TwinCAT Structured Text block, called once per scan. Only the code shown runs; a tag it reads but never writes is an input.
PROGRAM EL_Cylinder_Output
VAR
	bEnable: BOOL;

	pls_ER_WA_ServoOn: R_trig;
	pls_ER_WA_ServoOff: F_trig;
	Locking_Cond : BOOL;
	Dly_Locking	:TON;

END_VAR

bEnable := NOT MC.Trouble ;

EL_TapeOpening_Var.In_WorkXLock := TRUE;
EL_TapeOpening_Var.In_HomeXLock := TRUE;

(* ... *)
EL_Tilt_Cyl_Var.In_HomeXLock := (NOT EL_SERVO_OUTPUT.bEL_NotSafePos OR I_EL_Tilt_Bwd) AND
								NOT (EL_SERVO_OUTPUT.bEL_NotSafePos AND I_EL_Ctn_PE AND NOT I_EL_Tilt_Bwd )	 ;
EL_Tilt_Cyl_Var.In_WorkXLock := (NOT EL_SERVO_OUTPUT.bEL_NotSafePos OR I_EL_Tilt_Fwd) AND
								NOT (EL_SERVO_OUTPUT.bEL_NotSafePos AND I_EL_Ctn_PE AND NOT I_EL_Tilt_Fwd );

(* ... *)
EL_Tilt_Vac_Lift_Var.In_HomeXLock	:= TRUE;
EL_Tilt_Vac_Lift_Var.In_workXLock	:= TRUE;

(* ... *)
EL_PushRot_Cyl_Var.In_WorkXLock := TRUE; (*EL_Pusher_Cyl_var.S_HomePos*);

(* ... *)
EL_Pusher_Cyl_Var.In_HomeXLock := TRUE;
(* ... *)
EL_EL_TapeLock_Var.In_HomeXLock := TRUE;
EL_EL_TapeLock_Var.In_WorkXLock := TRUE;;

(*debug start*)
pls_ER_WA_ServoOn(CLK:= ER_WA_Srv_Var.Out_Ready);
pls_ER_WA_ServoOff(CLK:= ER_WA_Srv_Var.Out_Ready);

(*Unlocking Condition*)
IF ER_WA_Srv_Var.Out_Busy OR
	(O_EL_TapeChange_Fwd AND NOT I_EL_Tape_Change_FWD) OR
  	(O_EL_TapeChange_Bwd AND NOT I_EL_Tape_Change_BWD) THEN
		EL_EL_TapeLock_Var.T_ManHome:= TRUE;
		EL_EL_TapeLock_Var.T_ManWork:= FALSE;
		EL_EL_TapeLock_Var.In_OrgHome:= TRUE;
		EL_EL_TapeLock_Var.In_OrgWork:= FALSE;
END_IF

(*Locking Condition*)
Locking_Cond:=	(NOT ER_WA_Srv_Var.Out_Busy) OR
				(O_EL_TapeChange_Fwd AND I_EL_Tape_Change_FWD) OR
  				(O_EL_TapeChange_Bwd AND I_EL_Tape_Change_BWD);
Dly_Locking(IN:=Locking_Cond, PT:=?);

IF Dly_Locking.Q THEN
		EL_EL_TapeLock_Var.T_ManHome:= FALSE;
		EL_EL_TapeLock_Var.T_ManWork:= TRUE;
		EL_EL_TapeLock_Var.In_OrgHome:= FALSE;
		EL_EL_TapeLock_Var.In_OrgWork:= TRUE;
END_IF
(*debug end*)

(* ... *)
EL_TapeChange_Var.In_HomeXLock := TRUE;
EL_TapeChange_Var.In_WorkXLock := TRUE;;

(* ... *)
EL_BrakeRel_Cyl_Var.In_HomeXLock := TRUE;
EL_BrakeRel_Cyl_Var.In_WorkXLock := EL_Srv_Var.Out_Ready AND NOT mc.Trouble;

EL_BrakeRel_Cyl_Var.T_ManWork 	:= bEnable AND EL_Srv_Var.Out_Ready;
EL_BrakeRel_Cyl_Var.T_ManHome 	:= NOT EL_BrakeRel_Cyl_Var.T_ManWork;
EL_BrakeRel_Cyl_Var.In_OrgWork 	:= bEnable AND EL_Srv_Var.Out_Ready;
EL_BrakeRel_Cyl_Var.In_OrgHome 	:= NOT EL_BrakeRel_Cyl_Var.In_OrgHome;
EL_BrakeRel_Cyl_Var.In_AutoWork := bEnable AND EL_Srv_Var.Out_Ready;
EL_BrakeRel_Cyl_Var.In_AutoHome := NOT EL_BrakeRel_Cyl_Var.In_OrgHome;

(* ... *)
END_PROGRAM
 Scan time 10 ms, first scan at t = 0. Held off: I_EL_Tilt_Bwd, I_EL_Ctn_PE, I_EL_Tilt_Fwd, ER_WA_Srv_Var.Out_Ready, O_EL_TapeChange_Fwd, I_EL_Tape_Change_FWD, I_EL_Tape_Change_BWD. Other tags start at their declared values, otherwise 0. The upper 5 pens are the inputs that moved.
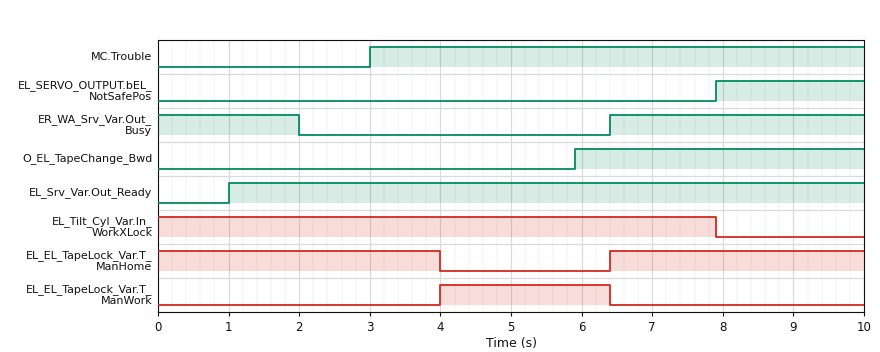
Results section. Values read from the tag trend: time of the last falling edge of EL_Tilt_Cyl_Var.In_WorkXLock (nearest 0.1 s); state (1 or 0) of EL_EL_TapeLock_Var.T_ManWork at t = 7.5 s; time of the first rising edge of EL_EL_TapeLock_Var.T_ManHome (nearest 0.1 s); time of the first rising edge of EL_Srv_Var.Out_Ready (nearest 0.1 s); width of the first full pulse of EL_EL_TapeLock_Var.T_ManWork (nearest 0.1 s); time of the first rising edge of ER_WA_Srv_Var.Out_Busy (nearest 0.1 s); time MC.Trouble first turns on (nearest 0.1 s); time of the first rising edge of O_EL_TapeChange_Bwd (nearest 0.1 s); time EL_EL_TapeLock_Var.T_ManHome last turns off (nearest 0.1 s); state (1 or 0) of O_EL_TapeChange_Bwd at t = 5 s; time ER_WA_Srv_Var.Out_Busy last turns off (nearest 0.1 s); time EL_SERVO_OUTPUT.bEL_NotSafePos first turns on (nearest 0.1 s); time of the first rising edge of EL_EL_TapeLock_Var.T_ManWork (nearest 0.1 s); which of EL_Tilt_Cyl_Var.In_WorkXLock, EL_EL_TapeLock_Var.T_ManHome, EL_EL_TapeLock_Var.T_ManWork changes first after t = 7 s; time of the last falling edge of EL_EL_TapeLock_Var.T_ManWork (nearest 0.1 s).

7.9 s
0
6.4 s
1.0 s
2.4 s
6.4 s
3.0 s
5.9 s
4.0 s
0
2.0 s
7.9 s
4.0 s
EL_Tilt_Cyl_Var.In_WorkXLock
6.4 s
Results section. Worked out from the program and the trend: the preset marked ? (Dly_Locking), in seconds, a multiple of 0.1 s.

2.0 s
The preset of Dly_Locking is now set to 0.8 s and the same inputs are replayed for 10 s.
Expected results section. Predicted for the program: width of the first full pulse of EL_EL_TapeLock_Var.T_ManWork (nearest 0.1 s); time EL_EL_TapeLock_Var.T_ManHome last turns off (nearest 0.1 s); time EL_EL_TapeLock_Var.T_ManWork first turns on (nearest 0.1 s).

3.6 s
2.8 s
2.8 s
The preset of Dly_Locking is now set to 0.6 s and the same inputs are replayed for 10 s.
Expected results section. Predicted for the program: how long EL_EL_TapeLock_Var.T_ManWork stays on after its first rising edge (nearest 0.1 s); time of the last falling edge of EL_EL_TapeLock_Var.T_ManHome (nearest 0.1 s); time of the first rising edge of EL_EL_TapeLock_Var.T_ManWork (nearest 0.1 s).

3.8 s
2.6 s
2.6 s
